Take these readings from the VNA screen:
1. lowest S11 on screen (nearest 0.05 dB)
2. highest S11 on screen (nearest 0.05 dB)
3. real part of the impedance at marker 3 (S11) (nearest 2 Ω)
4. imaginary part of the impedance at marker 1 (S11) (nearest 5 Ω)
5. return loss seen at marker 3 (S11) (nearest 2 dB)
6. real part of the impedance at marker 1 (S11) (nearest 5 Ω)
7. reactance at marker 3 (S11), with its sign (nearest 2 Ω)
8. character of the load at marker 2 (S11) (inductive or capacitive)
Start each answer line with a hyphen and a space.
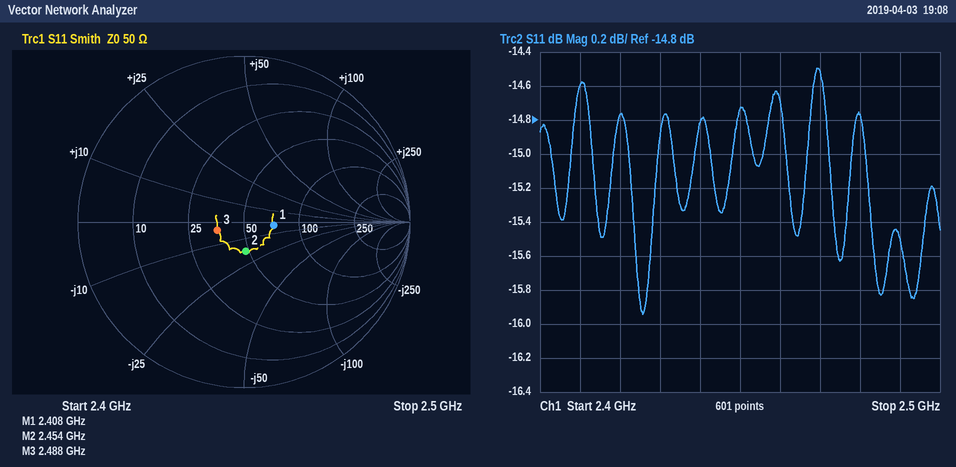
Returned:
- -15.95 dB
- -14.50 dB
- 36 Ω
- -5 Ω
- 16 dB
- 70 Ω
- -4 Ω
- capacitive
